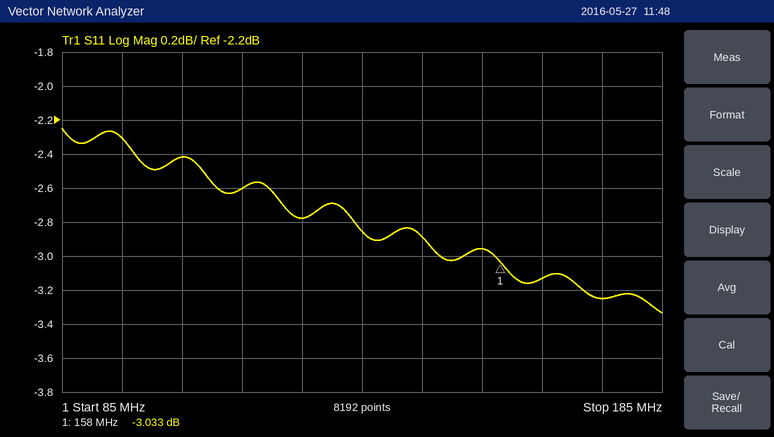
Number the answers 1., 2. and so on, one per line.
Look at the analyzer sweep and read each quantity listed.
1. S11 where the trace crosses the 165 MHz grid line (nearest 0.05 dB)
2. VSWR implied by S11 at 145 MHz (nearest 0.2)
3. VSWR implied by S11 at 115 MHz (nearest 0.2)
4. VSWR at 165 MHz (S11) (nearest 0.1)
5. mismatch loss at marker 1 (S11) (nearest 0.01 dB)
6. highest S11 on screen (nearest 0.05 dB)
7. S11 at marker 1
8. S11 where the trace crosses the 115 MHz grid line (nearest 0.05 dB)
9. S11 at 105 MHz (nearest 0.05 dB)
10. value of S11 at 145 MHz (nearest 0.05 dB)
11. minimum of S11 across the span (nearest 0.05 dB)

1. -3.15 dB
2. 6.0
3. 6.8
4. 5.6
5. 2.99 dB
6. -2.25 dB
7. -3.033 dB
8. -2.60 dB
9. -2.40 dB
10. -2.90 dB
11. -3.35 dB
